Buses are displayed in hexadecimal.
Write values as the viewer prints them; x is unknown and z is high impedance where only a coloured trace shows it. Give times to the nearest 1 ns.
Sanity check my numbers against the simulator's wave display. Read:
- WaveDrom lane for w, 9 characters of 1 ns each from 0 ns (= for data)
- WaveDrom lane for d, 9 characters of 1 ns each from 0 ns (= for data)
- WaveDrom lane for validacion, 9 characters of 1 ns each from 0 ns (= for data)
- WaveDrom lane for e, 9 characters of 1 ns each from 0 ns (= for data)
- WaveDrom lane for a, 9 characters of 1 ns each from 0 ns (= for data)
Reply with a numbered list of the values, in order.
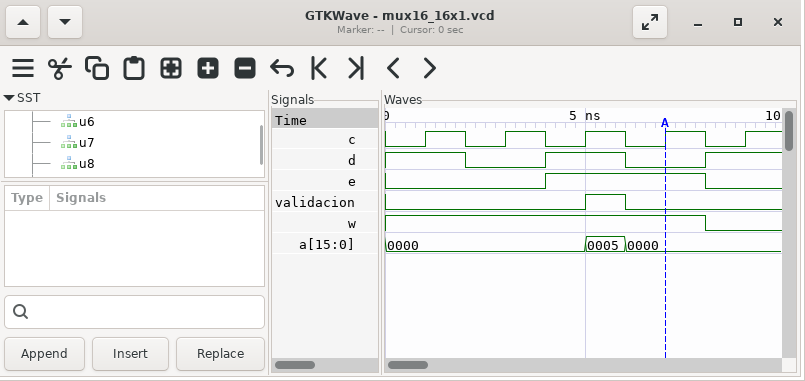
1. {name: 'w', wave: '1.......0'}
2. {name: 'd', wave: '1.0.1.0.1'}
3. {name: 'validacion', wave: '0....10..'}
4. {name: 'e', wave: '0...1...0'}
5. {name: 'a', wave: '=....==..', data: '0000 0005 0000'}
